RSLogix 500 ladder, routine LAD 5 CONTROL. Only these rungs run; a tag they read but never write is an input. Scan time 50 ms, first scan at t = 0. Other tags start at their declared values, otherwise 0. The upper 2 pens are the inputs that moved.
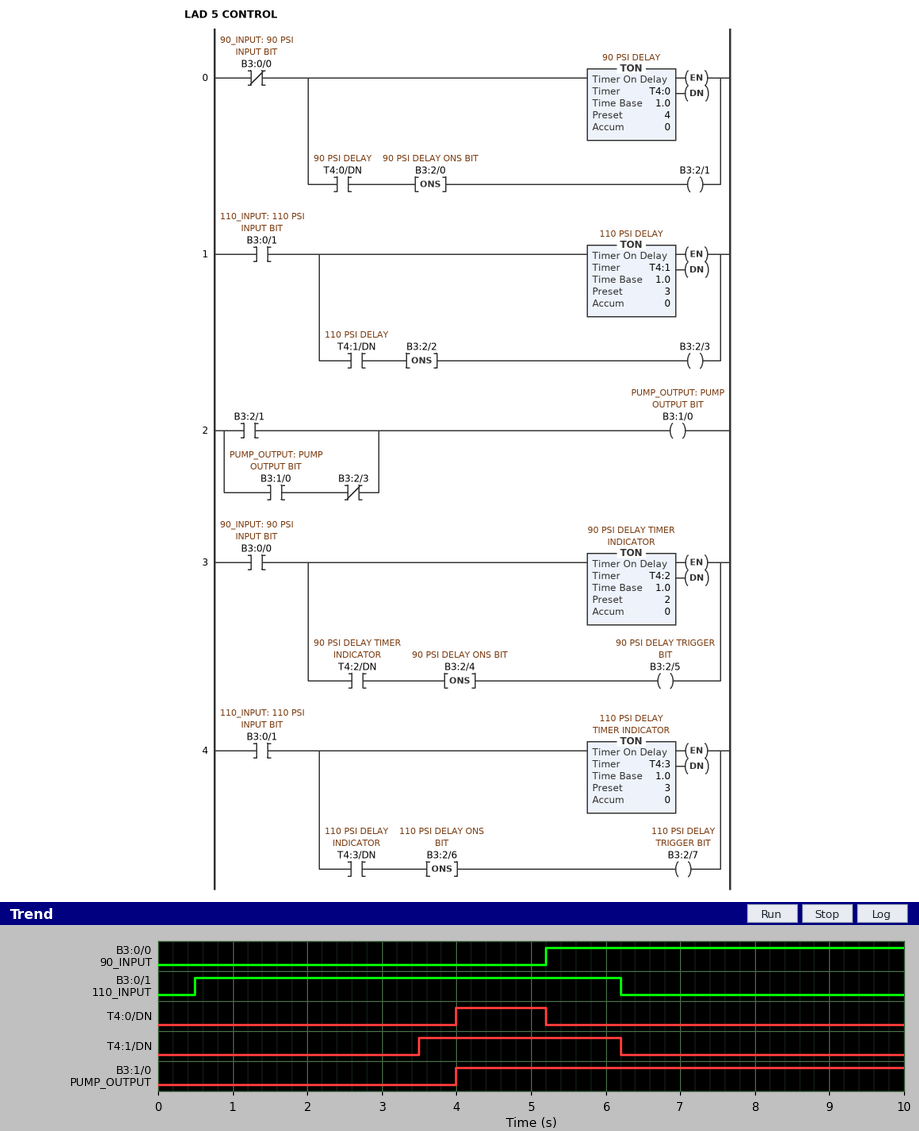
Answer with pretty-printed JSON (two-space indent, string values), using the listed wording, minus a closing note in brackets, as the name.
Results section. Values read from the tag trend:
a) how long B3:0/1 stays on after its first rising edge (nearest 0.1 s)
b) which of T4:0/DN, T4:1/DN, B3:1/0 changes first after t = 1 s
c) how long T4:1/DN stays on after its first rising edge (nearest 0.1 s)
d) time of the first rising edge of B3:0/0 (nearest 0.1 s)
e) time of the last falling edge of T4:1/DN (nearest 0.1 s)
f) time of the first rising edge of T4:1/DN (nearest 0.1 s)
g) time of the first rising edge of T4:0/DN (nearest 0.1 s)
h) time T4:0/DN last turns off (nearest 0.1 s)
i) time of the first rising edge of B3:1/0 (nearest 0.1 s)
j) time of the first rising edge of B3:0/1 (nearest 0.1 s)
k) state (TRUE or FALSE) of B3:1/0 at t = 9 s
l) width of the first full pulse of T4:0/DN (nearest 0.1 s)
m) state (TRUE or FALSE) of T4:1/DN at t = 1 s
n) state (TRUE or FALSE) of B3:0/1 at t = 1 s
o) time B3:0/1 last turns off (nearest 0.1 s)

{
  "how long B3:0/1 stays on after its first rising edge": "5.7 s",
  "which of T4:0/DN, T4:1/DN, B3:1/0 changes first after t = 1 s": "T4:1/DN",
  "how long T4:1/DN stays on after its first rising edge": "2.7 s",
  "time of the first rising edge of B3:0/0": "5.2 s",
  "time of the last falling edge of T4:1/DN": "6.2 s",
  "time of the first rising edge of T4:1/DN": "3.5 s",
  "time of the first rising edge of T4:0/DN": "4.0 s",
  "time T4:0/DN last turns off": "5.2 s",
  "time of the first rising edge of B3:1/0": "4.0 s",
  "time of the first rising edge of B3:0/1": "0.5 s",
  "state (TRUE or FALSE) of B3:1/0 at t = 9 s": "TRUE",
  "width of the first full pulse of T4:0/DN": "1.2 s",
  "state (TRUE or FALSE) of T4:1/DN at t = 1 s": "FALSE",
  "state (TRUE or FALSE) of B3:0/1 at t = 1 s": "TRUE",
  "time B3:0/1 last turns off": "6.2 s"
}
